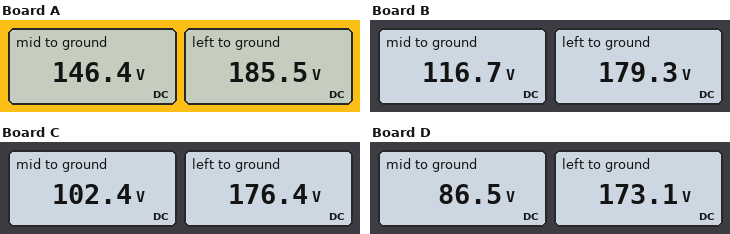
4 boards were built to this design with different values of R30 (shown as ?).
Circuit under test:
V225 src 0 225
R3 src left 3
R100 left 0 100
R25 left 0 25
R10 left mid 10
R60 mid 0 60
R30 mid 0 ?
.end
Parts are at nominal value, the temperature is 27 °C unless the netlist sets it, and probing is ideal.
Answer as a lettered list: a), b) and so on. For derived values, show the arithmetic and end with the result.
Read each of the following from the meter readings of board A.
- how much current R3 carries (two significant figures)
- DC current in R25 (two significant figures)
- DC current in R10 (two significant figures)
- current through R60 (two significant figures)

a) (225 V - 185.5 V) / 3 Ω = 13 A
b) (185.5 V) / 25 Ω = 7.4 A
c) (185.5 V - 146.4 V) / 10 Ω = 3.9 A
d) (146.4 V) / 60 Ω = 2.4 A
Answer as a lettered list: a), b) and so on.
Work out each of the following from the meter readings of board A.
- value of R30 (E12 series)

a) 100 Ω
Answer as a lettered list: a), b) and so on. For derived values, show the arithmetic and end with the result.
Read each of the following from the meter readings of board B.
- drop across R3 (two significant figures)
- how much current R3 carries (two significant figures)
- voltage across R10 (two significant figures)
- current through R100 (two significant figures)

a) 225 V - 179.3 V = 46 V
b) (225 V - 179.3 V) / 3 Ω = 15 A
c) 179.3 V - 116.7 V = 63 V
d) (179.3 V) / 100 Ω = 1.8 A
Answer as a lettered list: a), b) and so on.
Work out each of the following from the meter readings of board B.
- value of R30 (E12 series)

a) 27 Ω
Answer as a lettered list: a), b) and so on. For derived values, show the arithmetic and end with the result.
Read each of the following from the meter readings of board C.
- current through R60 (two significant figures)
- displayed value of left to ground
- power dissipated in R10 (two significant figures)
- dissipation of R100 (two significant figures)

a) (102.4 V) / 60 Ω = 1.7 A
b) 176.4 V
c) (176.4 V - 102.4 V)^2 / 10 Ω = 550 W
d) (176.4 V)^2 / 100 Ω = 310 W
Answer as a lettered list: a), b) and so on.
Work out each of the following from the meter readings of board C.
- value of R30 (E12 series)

a) 18 Ω
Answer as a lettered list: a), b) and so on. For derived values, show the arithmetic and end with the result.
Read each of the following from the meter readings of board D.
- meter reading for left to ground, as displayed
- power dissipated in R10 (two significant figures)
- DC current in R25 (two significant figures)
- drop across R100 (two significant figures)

a) 173.1 V
b) (173.1 V - 86.5 V)^2 / 10 Ω = 750 W
c) (173.1 V) / 25 Ω = 6.9 A
d) 173.1 V = 170 V
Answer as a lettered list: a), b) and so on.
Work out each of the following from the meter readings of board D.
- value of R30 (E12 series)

a) 12 Ω
